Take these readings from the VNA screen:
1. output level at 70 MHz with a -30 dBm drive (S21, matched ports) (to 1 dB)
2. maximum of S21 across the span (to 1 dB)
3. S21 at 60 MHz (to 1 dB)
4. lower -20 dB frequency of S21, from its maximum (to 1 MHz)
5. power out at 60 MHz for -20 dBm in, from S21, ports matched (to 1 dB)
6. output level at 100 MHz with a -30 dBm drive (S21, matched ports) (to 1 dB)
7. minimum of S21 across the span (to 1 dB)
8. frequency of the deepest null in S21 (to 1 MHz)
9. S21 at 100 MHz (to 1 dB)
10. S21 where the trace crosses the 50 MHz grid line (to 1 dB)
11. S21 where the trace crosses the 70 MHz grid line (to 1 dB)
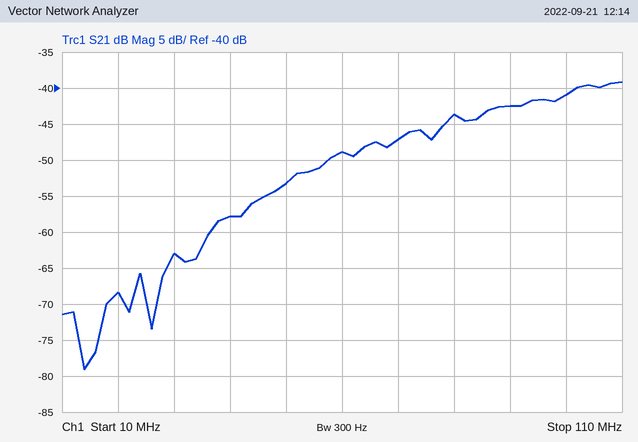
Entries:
-77 dBm
-39 dB
-49 dB
37 MHz
-69 dBm
-71 dBm
-79 dB
14 MHz
-41 dB
-53 dB
-47 dB
